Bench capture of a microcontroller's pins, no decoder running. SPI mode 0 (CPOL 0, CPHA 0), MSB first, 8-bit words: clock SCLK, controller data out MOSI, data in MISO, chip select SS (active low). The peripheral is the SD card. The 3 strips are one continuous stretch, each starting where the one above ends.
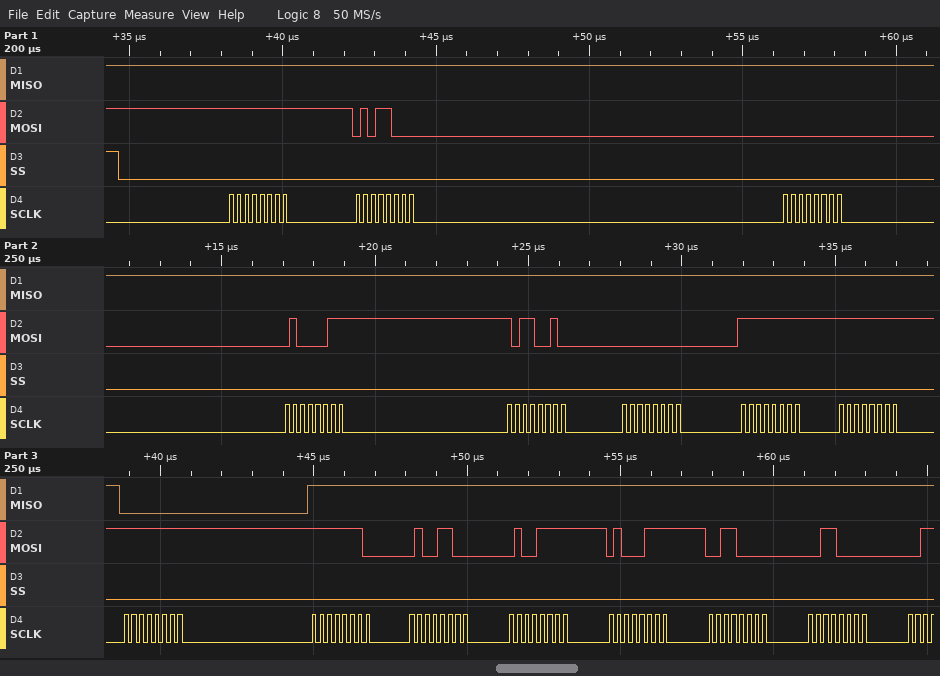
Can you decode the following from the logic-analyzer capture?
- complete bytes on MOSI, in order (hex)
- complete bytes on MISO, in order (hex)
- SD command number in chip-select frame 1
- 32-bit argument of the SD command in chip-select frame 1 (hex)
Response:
0xFF 0x58 0x00 0x43 0xB2 0x00 0xFF 0xFF 0xFF 0xFE 0x4C 0x4F 0x47 0x30 0x30
0xFF 0xFF 0xFF 0xFF 0xFF 0xFF 0xFF 0xFF 0x00 0xFF 0xFF 0xFF 0xFF 0xFF 0xFF
CMD24
0x0043B200
